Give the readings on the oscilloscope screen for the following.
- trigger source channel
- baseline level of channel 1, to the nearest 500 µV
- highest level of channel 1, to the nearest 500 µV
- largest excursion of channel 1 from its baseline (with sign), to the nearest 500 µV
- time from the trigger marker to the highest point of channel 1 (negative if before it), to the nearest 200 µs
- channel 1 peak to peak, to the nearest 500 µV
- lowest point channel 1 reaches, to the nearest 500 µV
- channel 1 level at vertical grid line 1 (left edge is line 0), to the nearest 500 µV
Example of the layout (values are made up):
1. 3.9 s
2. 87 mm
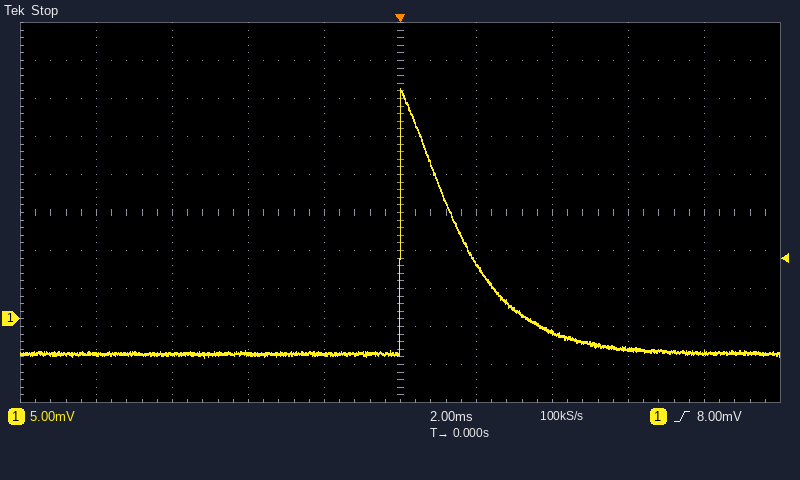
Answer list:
1. channel 1
2. -4.5 mV
3. 30.5 mV
4. +35.0 mV
5. 0.0 ms
6. 35.5 mV
7. -5.0 mV
8. -4.5 mV
